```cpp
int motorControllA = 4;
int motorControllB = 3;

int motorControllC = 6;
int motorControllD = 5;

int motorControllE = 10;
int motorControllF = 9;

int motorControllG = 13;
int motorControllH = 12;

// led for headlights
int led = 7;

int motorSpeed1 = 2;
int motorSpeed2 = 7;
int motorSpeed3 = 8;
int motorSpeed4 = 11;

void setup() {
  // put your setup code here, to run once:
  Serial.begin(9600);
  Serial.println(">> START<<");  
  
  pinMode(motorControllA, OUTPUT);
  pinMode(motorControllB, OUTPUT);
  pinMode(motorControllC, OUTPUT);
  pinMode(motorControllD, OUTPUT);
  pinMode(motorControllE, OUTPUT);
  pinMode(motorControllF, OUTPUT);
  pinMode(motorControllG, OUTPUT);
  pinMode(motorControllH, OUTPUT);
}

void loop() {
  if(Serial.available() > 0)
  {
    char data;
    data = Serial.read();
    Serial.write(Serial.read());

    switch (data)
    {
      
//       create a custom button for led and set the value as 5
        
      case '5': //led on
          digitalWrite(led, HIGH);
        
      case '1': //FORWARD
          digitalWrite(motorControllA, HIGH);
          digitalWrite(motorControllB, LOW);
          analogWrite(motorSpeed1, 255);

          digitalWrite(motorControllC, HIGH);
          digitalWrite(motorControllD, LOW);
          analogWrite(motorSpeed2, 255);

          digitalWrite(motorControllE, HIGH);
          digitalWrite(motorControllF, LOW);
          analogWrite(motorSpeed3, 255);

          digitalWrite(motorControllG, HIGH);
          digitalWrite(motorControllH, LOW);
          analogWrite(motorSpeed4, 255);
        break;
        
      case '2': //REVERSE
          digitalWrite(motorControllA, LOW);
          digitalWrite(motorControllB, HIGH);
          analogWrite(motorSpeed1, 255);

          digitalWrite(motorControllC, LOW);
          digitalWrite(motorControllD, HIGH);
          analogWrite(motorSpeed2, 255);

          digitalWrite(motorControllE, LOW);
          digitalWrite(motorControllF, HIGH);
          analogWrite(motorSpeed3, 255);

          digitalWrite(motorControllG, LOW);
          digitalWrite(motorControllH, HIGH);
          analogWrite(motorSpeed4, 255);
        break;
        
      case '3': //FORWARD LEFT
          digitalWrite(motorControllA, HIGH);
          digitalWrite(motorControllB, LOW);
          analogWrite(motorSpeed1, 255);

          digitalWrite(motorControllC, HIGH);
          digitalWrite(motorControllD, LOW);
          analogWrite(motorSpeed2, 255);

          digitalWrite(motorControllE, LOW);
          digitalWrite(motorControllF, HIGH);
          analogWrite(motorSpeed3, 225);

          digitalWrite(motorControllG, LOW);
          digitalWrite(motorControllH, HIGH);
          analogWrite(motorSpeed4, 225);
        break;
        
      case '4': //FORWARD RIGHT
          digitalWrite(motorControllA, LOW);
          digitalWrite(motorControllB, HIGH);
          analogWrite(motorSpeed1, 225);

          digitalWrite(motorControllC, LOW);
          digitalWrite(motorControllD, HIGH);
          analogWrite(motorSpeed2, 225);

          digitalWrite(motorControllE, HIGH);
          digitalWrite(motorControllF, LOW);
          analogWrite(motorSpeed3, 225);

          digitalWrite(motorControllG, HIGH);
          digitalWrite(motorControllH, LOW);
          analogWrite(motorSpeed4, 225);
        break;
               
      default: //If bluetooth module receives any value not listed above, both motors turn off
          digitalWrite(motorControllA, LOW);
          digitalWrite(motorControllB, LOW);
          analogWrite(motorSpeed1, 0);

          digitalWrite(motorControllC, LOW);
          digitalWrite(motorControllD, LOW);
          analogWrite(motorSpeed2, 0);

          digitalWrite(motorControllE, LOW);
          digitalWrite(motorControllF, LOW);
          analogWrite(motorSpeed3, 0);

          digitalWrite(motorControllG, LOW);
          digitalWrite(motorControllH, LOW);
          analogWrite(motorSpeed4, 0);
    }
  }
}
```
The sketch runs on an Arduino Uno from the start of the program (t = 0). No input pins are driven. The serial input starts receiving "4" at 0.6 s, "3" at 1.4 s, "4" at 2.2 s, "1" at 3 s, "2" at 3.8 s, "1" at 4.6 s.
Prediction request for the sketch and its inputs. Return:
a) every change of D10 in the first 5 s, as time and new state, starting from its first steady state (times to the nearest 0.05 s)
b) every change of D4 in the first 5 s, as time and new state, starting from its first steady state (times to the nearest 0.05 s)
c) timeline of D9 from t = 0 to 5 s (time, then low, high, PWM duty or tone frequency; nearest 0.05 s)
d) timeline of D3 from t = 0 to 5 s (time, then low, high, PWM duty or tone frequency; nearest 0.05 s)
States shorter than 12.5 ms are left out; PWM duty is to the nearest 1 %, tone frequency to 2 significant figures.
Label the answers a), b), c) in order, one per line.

a) 0 s low; 0.6 s high; 1.4 s low; 2.2 s high; 3.8 s low; 4.6 s high
b) 0 s low; 1.4 s high; 2.2 s low; 3 s high; 3.8 s low; 4.6 s high
c) 0 s low; 1.4 s high; 2.2 s low; 3.8 s high; 4.6 s low
d) 0 s low; 0.6 s high; 1.4 s low; 2.2 s high; 3 s low; 3.8 s high; 4.6 s low
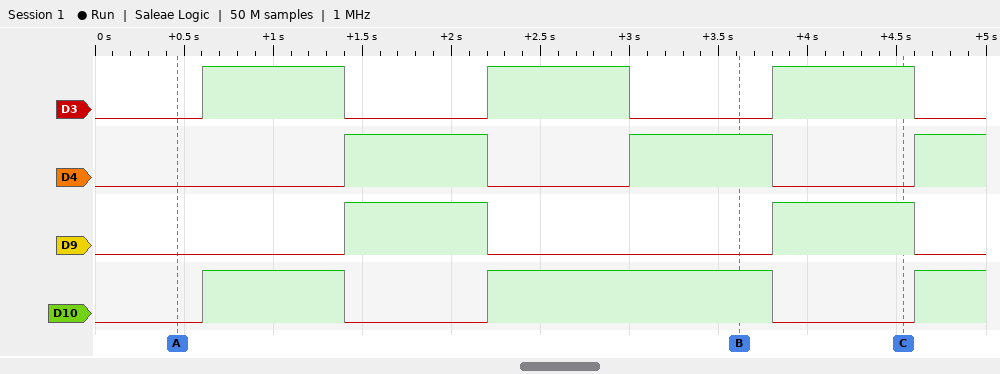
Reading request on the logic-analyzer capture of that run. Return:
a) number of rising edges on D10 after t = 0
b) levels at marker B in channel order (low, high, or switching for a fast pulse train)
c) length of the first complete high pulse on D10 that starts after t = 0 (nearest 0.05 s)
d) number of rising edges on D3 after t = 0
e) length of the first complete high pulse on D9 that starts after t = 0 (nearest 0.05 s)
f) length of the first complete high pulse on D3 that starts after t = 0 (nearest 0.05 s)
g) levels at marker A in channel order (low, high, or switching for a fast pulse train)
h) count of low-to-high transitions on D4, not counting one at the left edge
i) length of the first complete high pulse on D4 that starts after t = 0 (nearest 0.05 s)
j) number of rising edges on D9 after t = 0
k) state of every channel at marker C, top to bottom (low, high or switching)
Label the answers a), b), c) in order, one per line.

a) 3
b) D3 low, D4 high, D9 low, D10 high
c) 0.80 s
d) 3
e) 0.80 s
f) 0.80 s
g) D3 low, D4 low, D9 low, D10 low
h) 3
i) 0.80 s
j) 2
k) D3 high, D4 low, D9 high, D10 low
